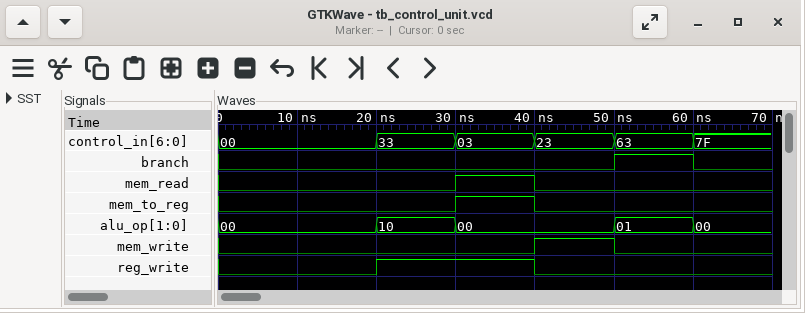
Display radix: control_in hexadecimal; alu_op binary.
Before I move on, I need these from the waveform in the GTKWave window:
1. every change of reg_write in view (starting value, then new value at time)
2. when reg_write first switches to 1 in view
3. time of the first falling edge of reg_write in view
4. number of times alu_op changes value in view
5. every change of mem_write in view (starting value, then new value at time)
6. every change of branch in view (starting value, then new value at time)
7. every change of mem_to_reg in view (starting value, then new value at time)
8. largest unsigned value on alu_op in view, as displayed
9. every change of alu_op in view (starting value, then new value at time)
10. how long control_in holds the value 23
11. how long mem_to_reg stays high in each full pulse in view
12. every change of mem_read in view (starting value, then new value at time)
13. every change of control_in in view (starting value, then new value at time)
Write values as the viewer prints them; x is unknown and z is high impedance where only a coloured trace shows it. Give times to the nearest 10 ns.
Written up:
0, 1 at 20 ns, 0 at 40 ns
20 ns
40 ns
4
0, 1 at 40 ns, 0 at 50 ns
0, 1 at 50 ns, 0 at 60 ns
0, 1 at 30 ns, 0 at 40 ns
10
00, 10 at 20 ns, 00 at 30 ns, 01 at 50 ns, 00 at 60 ns
10 ns
10 ns
0, 1 at 30 ns, 0 at 40 ns
00, 33 at 20 ns, 03 at 30 ns, 23 at 40 ns, 63 at 50 ns, 7F at 60 ns
